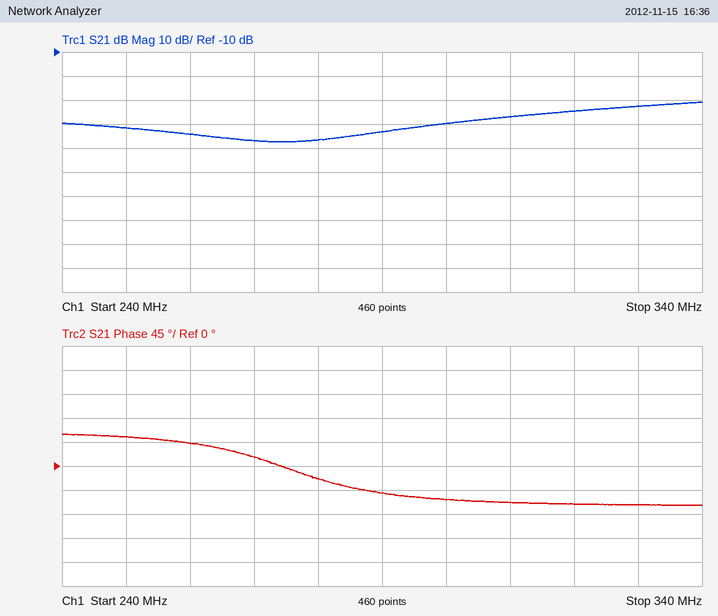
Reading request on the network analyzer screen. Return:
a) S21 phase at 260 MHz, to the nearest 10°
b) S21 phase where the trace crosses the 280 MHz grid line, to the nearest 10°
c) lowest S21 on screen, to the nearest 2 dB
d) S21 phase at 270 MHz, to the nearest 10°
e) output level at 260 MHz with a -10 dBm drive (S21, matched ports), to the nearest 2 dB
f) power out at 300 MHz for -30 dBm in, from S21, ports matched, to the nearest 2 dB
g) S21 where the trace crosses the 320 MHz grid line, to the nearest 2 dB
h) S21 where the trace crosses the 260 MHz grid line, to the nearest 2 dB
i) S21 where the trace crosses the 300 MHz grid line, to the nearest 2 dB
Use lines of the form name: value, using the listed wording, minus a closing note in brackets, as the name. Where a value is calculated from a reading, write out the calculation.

S21 phase at 260 MHz, to the nearest 10°: 40°
S21 phase where the trace crosses the 280 MHz grid line, to the nearest 10°: -20°
lowest S21 on screen, to the nearest 2 dB: -48 dB
S21 phase at 270 MHz, to the nearest 10°: 20°
output level at 260 MHz with a -10 dBm drive (S21, matched ports), to the nearest 2 dB: -10 dBm + (-44 dB) = -54 dBm
power out at 300 MHz for -30 dBm in, from S21, ports matched, to the nearest 2 dB: -30 dBm + (-40 dB) = -70 dBm
S21 where the trace crosses the 320 MHz grid line, to the nearest 2 dB: -34 dB
S21 where the trace crosses the 260 MHz grid line, to the nearest 2 dB: -44 dB
S21 where the trace crosses the 300 MHz grid line, to the nearest 2 dB: -40 dB
